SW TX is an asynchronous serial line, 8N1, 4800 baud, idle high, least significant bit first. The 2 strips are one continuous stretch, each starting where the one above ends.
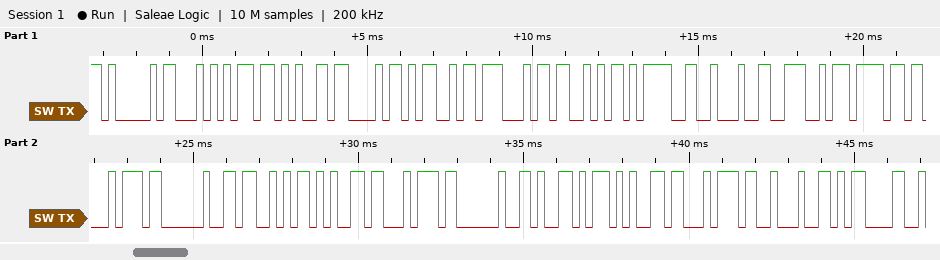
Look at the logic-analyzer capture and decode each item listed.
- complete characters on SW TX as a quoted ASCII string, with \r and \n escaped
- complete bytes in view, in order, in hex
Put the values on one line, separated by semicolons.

"AT+CMGS=\"Not Set Yet\"\r"; 41 54 2B 43 4D 47 53 3D 22 4E 6F 74 20 53 65 74 20 59 65 74 22 0D
